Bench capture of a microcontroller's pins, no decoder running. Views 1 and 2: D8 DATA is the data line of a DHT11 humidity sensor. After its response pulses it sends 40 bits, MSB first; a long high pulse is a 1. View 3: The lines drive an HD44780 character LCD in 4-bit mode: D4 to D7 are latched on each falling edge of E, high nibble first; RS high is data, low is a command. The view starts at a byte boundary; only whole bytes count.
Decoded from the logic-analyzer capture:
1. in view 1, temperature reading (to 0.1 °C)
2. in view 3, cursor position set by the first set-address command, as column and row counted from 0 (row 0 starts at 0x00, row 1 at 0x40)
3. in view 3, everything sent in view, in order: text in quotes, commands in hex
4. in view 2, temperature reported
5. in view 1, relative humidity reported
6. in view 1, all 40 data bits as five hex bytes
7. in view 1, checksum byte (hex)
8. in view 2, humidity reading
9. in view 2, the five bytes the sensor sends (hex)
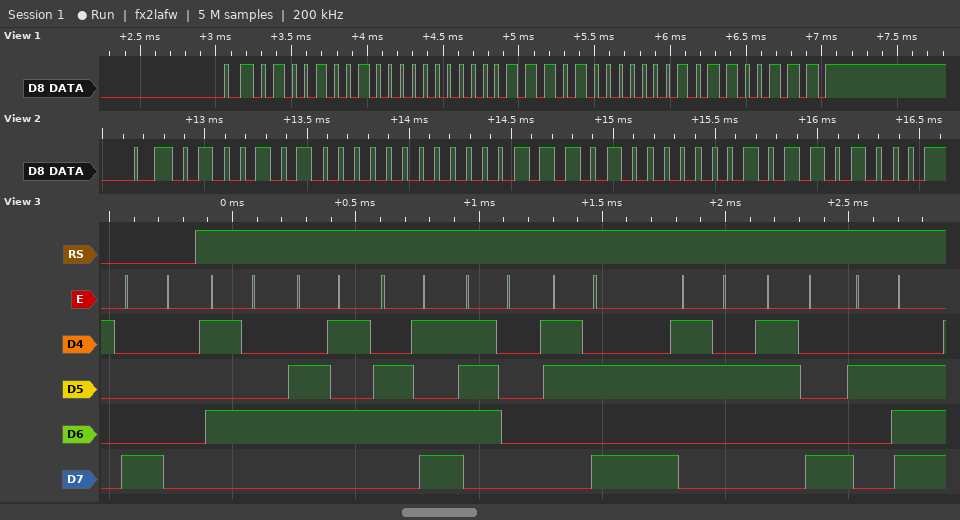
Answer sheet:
29.1 °C
column 0, row 0
0x80 "Temp:28."
29.1 °C
73 %
49 00 1D 01 67
0x67
74 %
4A 00 1D 01 68
